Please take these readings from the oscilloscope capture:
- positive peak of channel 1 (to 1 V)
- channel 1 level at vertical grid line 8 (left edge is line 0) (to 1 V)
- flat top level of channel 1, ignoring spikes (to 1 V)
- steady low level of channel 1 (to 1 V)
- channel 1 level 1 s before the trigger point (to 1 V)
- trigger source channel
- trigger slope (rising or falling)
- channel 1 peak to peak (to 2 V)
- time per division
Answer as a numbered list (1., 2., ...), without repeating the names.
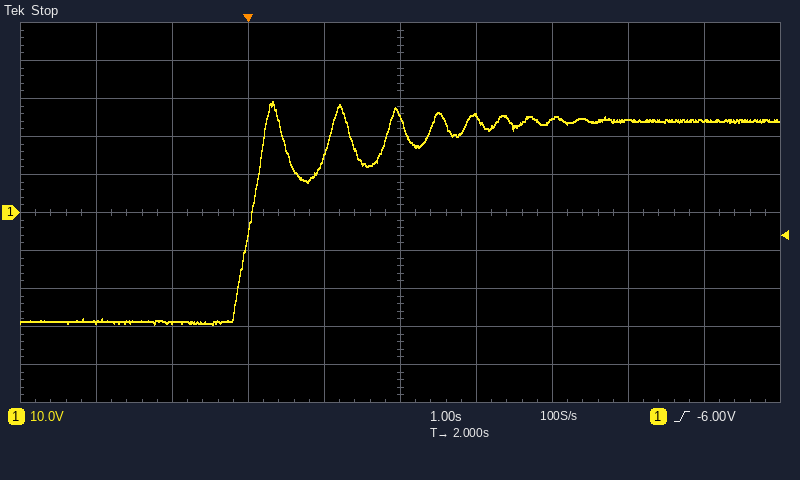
1. 29 V
2. 24 V
3. 24 V
4. -29 V
5. -29 V
6. channel 1
7. rising
8. 58 V
9. 1 s
